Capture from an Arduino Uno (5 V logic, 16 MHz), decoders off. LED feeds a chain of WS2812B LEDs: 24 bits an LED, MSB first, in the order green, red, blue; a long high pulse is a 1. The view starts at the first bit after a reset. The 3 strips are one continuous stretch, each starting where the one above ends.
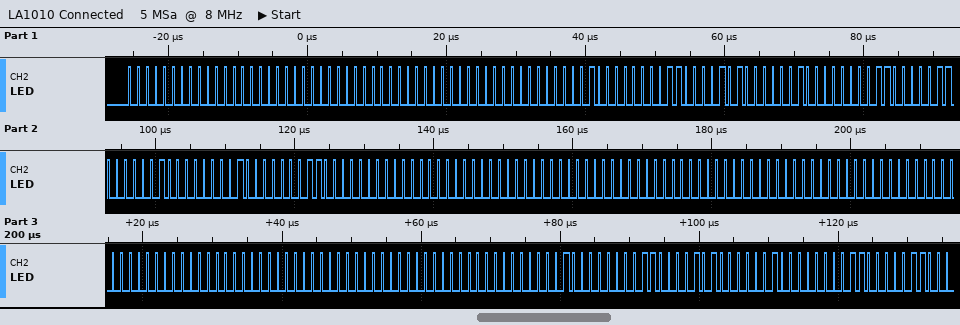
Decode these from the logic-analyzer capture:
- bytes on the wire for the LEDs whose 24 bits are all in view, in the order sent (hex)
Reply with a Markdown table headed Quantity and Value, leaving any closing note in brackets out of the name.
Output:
| Quantity | Value |
|---|---|
| bytes on the wire for the LEDs whose 24 bits are all in view, in the order sent | 00 00 00 00 00 00 04 03 0A 04 03 06 04 02 03 00 00 00 00 00 00 00 00 00 00 00 00 00 00 00 04 03 0A 04 03 06 |
